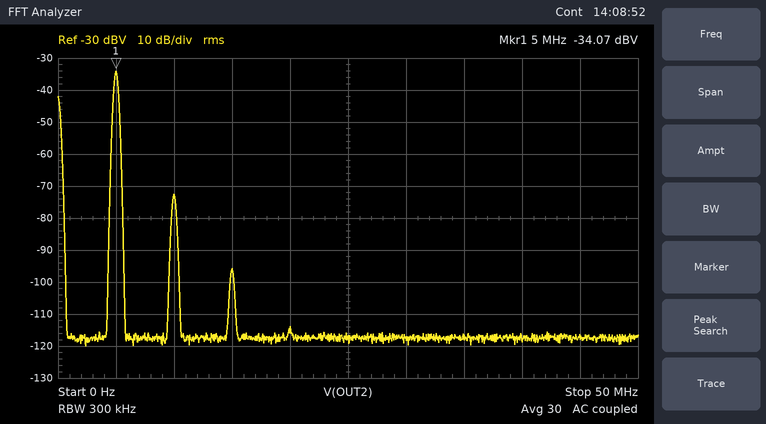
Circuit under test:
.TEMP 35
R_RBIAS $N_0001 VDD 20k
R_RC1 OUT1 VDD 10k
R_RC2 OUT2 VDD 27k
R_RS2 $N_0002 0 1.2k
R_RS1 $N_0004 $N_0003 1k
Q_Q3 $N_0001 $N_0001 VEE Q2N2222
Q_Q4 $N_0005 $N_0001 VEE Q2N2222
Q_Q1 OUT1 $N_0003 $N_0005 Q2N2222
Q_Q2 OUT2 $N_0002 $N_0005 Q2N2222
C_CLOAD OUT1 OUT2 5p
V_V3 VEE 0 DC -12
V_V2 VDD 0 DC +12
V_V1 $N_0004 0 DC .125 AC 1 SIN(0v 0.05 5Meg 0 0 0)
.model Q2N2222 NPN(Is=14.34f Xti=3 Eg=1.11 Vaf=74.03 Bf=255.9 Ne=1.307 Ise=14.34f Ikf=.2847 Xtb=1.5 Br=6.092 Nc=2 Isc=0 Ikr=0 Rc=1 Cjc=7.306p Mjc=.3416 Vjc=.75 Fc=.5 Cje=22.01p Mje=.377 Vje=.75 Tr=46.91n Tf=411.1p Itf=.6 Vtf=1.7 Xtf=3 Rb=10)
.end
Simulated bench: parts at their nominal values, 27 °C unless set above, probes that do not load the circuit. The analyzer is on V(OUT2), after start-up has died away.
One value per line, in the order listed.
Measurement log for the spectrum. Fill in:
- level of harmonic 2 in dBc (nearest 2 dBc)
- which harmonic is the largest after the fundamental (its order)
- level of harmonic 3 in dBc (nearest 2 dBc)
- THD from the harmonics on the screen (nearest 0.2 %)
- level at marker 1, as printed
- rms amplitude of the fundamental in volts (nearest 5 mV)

-38 dBc
2
-62 dBc
1.2 %
-34.07 dBV
20 mV
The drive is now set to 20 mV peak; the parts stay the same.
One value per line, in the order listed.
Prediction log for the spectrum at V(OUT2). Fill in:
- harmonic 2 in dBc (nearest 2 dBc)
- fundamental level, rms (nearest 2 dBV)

-46 dBc
-42 dBV
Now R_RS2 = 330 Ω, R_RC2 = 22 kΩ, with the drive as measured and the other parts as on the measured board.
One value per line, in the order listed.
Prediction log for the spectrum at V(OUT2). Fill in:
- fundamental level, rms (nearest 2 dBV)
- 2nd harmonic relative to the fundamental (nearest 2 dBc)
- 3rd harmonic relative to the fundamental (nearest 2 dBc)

-40 dBV
-28 dBc
-48 dBc
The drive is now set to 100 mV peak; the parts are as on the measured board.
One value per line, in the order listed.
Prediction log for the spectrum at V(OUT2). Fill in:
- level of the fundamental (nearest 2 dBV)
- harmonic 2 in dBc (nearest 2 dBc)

-28 dBV
-32 dBc
